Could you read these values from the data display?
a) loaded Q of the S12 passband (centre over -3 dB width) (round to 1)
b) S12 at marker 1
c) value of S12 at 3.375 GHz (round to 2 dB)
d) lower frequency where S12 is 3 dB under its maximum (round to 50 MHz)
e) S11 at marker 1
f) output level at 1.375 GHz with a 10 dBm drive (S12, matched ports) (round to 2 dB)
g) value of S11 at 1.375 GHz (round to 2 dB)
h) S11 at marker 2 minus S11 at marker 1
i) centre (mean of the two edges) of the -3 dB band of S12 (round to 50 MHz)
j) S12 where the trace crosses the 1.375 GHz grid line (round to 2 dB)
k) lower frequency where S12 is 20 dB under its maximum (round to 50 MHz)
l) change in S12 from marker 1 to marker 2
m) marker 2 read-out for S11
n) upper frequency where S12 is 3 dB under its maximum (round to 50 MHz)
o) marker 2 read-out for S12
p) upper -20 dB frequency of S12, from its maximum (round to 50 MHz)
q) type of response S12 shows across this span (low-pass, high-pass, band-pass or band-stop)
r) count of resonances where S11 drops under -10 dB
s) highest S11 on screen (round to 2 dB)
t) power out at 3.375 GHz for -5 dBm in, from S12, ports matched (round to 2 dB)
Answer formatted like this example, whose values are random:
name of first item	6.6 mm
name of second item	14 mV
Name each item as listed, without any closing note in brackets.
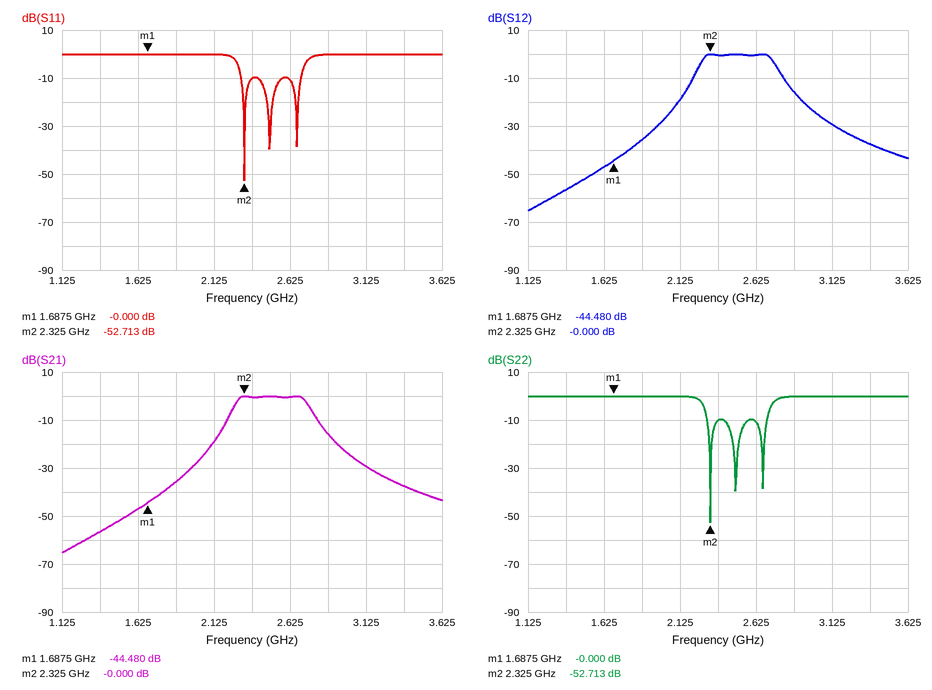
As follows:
loaded Q of the S12 passband (centre over -3 dB width)	5
S12 at marker 1	-44.480 dB
value of S12 at 3.375 GHz	-38 dB
lower frequency where S12 is 3 dB under its maximum	2.25 GHz
S11 at marker 1	-0.000 dB
output level at 1.375 GHz with a 10 dBm drive (S12, matched ports)	-46 dBm
value of S11 at 1.375 GHz	0 dB
S11 at marker 2 minus S11 at marker 1	-52.713 dB
centre (mean of the two edges) of the -3 dB band of S12	2.50 GHz
S12 where the trace crosses the 1.375 GHz grid line	-56 dB
lower frequency where S12 is 20 dB under its maximum	2.10 GHz
change in S12 from marker 1 to marker 2	44.480 dB
marker 2 read-out for S11	-52.713 dB
upper frequency where S12 is 3 dB under its maximum	2.75 GHz
marker 2 read-out for S12	-0.000 dB
upper -20 dB frequency of S12, from its maximum	2.95 GHz
type of response S12 shows across this span	band-pass
count of resonances where S11 drops under -10 dB	3
highest S11 on screen	0 dB
power out at 3.375 GHz for -5 dBm in, from S12, ports matched	-42 dBm
